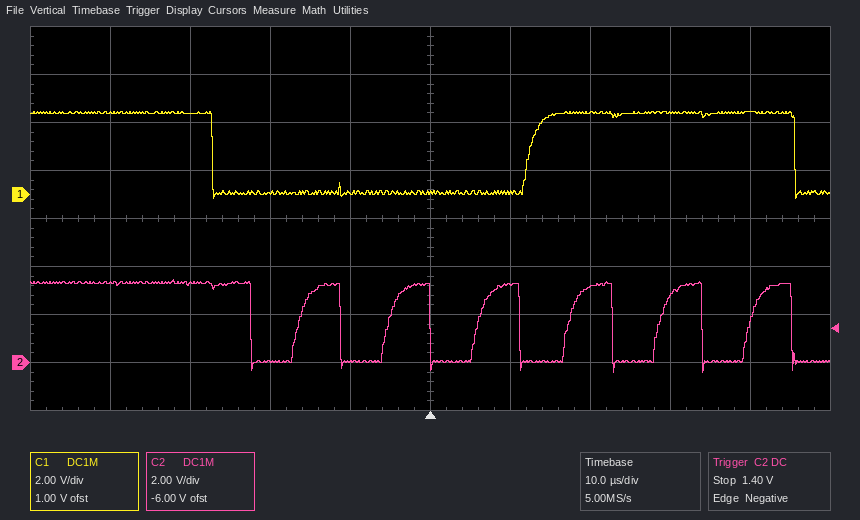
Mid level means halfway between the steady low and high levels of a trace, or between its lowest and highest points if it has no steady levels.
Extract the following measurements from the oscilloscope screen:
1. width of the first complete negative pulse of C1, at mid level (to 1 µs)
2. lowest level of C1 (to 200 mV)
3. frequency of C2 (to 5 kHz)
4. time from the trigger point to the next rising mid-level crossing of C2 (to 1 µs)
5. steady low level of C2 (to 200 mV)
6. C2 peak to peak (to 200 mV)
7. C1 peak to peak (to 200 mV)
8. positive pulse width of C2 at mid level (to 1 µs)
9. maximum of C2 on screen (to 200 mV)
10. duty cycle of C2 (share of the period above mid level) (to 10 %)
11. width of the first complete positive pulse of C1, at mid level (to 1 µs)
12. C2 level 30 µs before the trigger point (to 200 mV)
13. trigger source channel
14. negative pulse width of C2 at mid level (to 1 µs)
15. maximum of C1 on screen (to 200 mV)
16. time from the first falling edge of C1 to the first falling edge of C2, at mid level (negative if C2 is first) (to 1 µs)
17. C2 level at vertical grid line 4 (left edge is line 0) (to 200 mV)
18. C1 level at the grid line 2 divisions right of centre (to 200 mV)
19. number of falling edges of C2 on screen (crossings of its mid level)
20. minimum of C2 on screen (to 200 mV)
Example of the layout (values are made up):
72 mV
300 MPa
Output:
40 µs
-200 mV
90 kHz
6 µs
0.0 V
3.8 V
3.6 V
5 µs
3.4 V
50 %
33 µs
3.2 V
C2
6 µs
3.4 V
+5 µs
0.0 V
3.4 V
7
-400 mV
